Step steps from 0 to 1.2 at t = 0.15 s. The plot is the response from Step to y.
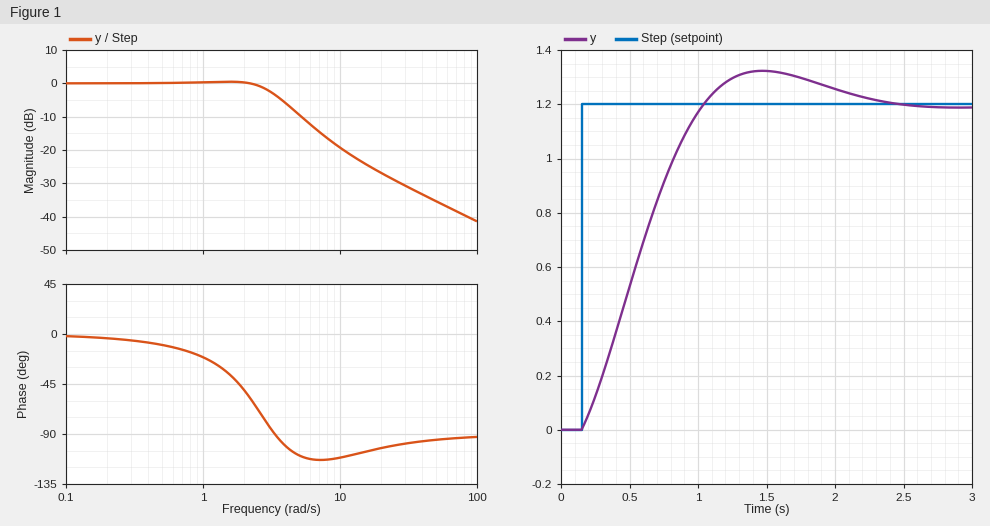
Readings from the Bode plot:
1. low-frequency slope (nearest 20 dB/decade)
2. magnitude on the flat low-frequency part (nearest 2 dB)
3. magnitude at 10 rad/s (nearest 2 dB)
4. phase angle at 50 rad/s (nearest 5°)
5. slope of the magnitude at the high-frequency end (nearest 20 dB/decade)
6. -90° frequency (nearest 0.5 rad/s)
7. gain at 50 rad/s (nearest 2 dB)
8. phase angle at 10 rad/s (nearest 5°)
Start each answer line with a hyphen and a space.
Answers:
- 0 dB/decade
- 0 dB
- -20 dB
- -95°
- -20 dB/decade
- 3.5 rad/s
- -36 dB
- -110°
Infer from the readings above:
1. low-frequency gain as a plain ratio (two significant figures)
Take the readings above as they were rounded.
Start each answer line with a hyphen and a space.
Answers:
- 1.0
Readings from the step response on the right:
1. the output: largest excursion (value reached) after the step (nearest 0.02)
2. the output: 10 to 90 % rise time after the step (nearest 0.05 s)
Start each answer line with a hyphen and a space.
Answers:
- 1.32
- 0.65 s
